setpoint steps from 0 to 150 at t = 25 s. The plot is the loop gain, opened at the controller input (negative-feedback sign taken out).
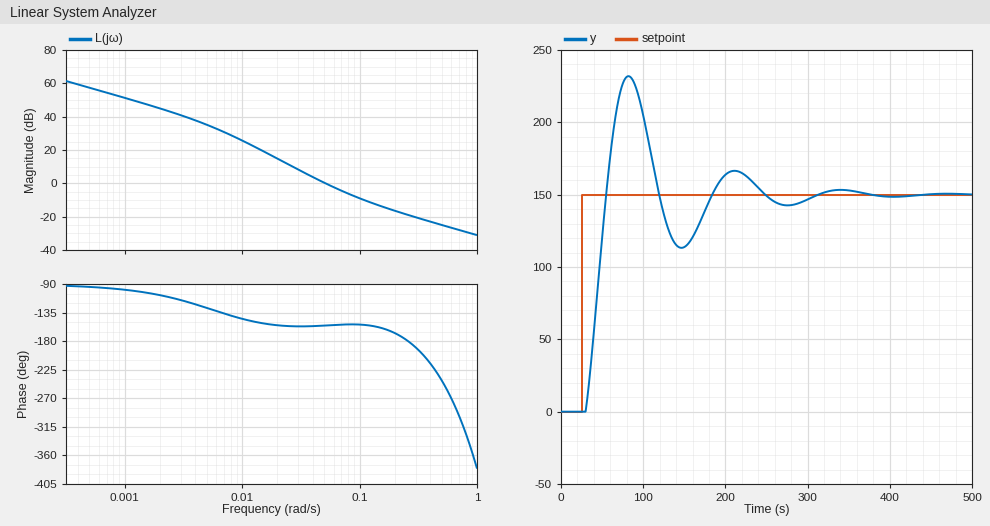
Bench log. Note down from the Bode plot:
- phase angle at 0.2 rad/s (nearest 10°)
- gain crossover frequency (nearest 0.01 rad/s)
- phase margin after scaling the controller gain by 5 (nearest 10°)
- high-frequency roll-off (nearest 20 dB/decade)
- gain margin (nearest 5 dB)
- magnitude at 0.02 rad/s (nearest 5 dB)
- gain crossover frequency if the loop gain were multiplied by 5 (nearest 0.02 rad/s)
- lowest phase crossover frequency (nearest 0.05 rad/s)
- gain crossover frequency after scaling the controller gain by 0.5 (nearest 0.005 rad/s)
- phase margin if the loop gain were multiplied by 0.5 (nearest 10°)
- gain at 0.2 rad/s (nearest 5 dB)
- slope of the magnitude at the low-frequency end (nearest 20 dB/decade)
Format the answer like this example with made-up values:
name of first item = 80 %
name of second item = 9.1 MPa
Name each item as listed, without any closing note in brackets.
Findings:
phase angle at 0.2 rad/s = -170°
gain crossover frequency = 0.05 rad/s
phase margin after scaling the controller gain by 5 = 20°
high-frequency roll-off = -20 dB/decade
gain margin = 20 dB
magnitude at 0.02 rad/s = 15 dB
gain crossover frequency if the loop gain were multiplied by 5 = 0.16 rad/s
lowest phase crossover frequency = 0.25 rad/s
gain crossover frequency after scaling the controller gain by 0.5 = 0.035 rad/s
phase margin if the loop gain were multiplied by 0.5 = 20°
gain at 0.2 rad/s = -15 dB
slope of the magnitude at the low-frequency end = -20 dB/decade
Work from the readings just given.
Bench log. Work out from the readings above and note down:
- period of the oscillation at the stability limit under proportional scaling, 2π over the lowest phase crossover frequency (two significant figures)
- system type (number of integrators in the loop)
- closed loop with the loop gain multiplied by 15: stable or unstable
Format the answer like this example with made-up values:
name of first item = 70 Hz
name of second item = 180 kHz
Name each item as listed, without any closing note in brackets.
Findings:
period of the oscillation at the stability limit under proportional scaling, 2π over the lowest phase crossover frequency = 25 s
system type = 1
closed loop with the loop gain multiplied by 15: stable or unstable = unstable
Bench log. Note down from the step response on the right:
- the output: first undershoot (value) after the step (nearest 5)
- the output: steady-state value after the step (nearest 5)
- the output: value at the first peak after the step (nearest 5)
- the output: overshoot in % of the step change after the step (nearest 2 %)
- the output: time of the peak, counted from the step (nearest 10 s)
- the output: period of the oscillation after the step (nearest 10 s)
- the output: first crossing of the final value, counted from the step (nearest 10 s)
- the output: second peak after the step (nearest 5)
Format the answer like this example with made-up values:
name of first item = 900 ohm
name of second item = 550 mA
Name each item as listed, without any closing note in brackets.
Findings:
the output: first undershoot (value) after the step = 115
the output: steady-state value after the step = 150
the output: value at the first peak after the step = 230
the output: overshoot in % of the step change after the step = 54 %
the output: time of the peak, counted from the step = 60 s
the output: period of the oscillation after the step = 130 s
the output: first crossing of the final value, counted from the step = 30 s
the output: second peak after the step = 165
